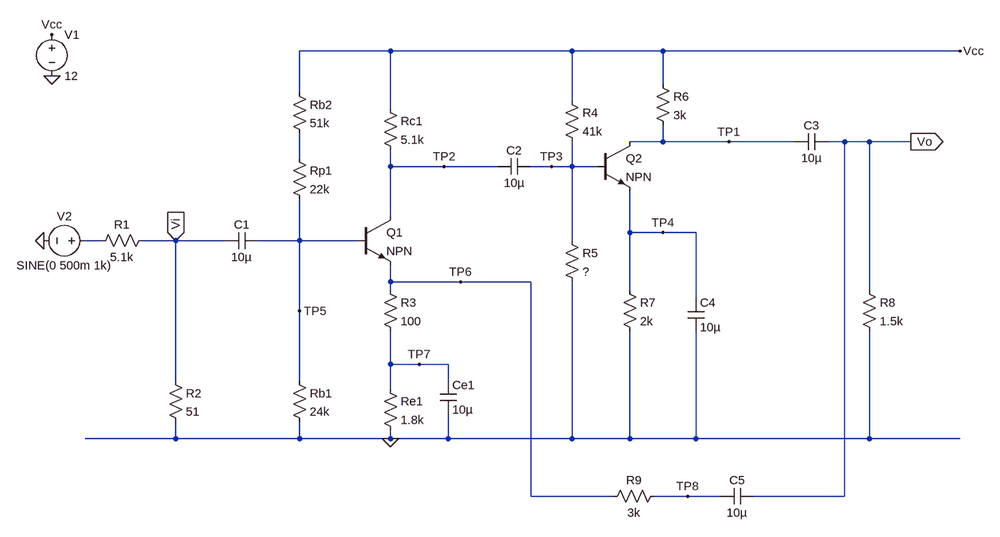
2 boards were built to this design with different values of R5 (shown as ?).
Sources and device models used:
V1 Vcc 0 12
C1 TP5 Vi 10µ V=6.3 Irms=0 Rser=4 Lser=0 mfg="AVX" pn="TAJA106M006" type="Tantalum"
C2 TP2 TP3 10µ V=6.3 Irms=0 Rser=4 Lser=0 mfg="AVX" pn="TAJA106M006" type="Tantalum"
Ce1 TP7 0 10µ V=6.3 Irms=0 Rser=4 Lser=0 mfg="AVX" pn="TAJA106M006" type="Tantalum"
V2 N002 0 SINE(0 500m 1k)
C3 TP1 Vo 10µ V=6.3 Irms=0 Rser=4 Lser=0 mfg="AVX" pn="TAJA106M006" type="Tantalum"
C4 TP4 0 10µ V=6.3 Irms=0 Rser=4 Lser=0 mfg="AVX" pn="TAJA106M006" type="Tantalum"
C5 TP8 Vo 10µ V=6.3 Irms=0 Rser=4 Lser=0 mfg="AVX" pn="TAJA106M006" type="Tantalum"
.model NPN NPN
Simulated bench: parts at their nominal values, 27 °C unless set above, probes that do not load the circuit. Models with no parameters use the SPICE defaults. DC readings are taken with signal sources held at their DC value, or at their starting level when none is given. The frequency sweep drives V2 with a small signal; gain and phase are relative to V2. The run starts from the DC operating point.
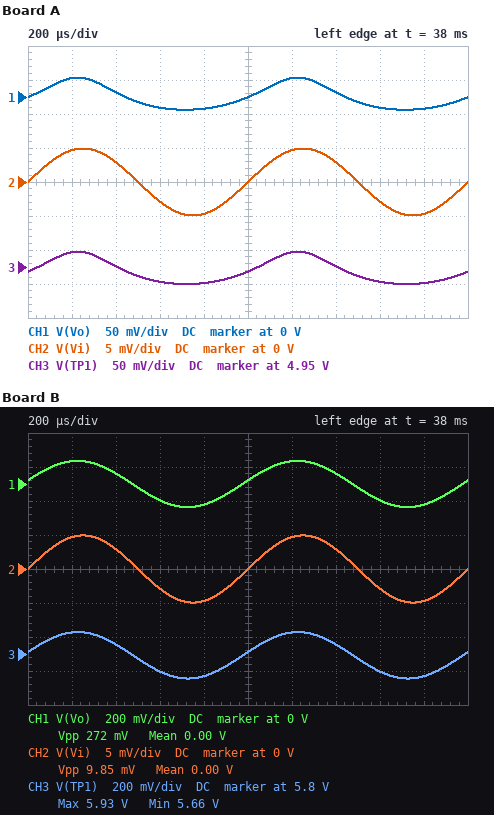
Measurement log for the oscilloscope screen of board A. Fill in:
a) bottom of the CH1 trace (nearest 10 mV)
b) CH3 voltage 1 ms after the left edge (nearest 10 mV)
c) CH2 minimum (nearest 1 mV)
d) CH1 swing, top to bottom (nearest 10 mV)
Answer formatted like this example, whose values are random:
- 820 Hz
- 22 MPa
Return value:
- -20 mV
- 4.94 V
- -5 mV
- 50 mV
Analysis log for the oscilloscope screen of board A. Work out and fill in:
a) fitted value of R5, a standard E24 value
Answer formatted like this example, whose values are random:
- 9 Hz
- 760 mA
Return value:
- 62 kΩ
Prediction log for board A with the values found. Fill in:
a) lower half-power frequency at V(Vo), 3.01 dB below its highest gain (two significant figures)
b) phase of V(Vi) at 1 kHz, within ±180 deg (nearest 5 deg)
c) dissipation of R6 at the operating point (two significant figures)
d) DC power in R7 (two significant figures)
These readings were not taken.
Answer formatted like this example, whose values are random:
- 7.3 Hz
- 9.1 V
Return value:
- 150 Hz
- 0 deg
- 17 mW
- 12 mW
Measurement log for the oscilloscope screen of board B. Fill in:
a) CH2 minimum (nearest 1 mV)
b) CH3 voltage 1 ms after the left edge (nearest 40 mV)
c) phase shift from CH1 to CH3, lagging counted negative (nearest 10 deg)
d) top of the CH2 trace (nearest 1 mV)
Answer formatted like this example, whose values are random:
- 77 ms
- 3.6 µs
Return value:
- -5 mV
- 5.80 V
- 0 deg
- 5 mV
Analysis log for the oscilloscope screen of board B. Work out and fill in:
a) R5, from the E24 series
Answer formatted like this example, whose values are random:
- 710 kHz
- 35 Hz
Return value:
- 33 kΩ
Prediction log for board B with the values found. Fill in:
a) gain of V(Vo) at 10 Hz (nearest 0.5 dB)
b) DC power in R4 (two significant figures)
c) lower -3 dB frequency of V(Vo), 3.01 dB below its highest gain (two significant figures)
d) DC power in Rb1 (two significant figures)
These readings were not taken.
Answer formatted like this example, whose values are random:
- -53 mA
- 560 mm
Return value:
- -34.0 dB
- 1.2 mW
- 160 Hz
- 320 µW
